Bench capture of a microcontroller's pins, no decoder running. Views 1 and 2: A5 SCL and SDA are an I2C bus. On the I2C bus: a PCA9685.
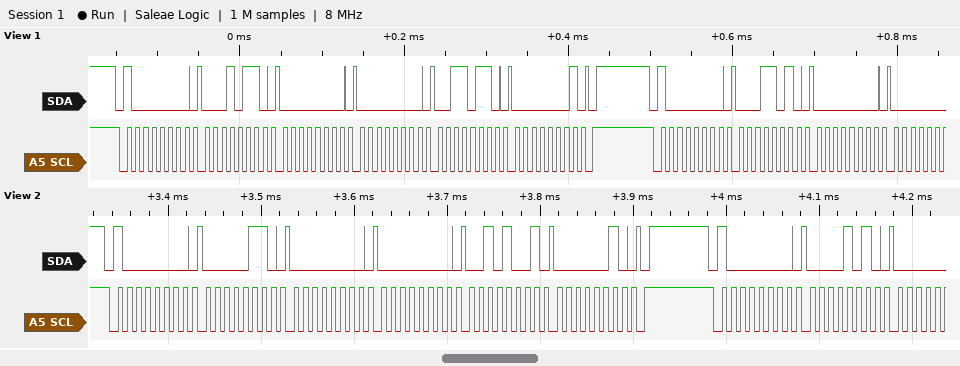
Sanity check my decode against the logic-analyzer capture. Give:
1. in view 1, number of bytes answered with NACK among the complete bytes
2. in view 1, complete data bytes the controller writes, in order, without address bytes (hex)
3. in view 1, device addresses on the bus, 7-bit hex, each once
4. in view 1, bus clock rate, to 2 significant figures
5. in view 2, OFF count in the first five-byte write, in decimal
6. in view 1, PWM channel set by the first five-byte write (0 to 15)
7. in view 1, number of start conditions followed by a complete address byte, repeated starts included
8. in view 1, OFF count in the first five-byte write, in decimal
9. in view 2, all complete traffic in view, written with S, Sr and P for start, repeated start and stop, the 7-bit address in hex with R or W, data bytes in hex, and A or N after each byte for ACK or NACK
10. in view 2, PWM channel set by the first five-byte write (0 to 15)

0
16 00 00 36 01 1A 00
0x40
100 kHz
553
4
2
310
S 40W A 06 A 00 A 00 A 29 A 02 A P S 40W A 0A A
0
